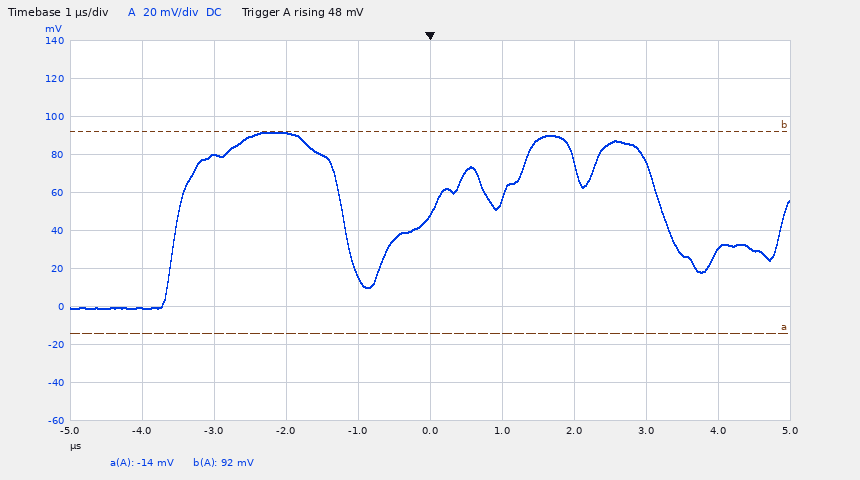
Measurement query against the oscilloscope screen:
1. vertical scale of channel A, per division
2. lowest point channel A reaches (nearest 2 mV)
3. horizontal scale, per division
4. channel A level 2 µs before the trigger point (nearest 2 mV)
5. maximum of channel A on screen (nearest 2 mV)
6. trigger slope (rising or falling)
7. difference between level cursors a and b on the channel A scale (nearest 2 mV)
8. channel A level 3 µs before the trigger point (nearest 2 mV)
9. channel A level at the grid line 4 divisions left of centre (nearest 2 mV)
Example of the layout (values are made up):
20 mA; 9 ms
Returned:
20 mV; -2 mV; 1 µs; 92 mV; 92 mV; rising; 106 mV; 80 mV; 0 mV
